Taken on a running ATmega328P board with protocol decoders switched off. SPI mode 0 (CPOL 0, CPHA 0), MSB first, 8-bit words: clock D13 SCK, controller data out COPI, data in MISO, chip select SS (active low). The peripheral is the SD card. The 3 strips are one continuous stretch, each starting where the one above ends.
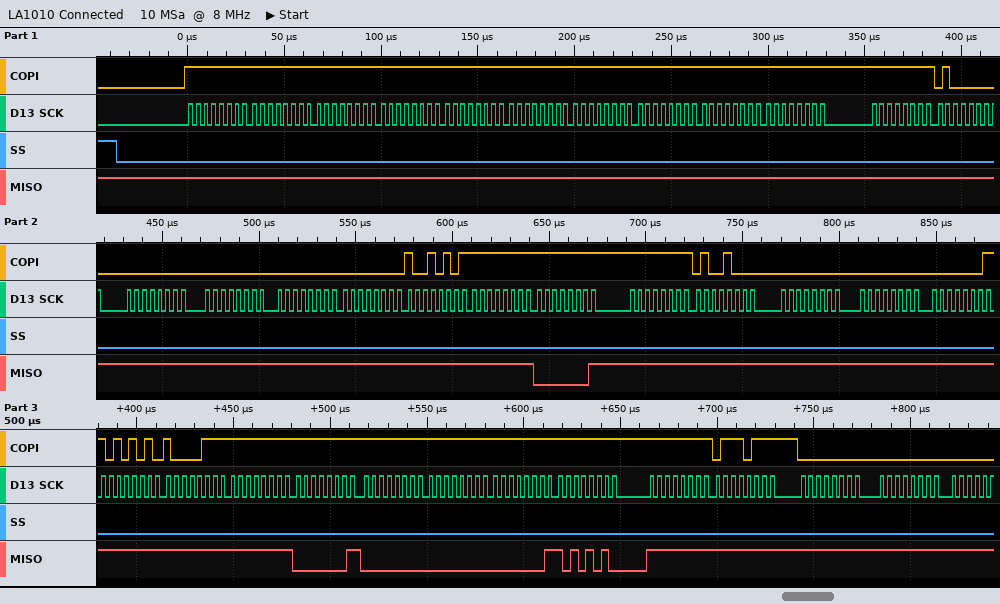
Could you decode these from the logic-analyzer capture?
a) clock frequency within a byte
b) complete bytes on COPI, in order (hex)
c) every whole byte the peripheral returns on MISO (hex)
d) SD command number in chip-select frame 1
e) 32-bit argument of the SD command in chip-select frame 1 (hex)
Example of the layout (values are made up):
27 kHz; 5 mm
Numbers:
250 kHz; FF FF FF FF FF FF FF FF FF FF FF 40 00 00 00 00 95 FF FF FF 48 00 00 01 AA 87 FF FF FF FF FF FF FF 77 00 00; FF FF FF FF FF FF FF FF FF FF FF FF FF FF FF FF FF FF 01 FF FF FF FF FF FF FF FF 01 00 00 01 AA FF FF FF FF; CMD0; 0x00000000
